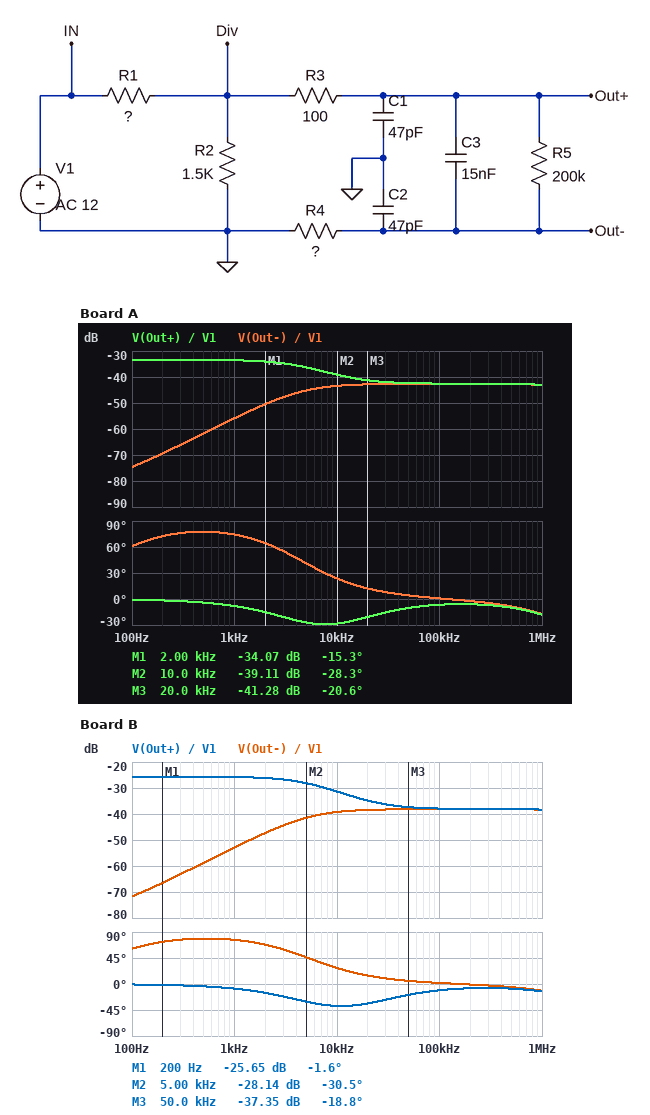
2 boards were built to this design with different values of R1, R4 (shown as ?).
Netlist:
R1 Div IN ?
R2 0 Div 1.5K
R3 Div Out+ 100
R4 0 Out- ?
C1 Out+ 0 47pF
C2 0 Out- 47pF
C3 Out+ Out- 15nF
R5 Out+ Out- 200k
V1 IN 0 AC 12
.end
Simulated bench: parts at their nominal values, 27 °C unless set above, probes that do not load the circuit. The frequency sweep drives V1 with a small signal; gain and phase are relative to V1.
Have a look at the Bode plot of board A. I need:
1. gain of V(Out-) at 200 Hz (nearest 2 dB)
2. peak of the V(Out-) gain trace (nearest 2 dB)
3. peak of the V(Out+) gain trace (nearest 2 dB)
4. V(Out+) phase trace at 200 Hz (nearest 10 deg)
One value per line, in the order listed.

-70 dB
-42 dB
-34 dB
0 deg
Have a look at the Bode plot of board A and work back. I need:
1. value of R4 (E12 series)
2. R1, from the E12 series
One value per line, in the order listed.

820 Ω
68 kΩ
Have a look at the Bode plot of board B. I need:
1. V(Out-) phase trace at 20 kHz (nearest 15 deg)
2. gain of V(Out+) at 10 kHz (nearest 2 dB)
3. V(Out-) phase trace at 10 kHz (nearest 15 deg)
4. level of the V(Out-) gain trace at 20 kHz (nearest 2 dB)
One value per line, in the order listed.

15 deg
-32 dB
30 deg
-38 dB
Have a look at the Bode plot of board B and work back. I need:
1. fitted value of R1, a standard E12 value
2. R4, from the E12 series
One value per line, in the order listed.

27 kΩ
470 Ω
